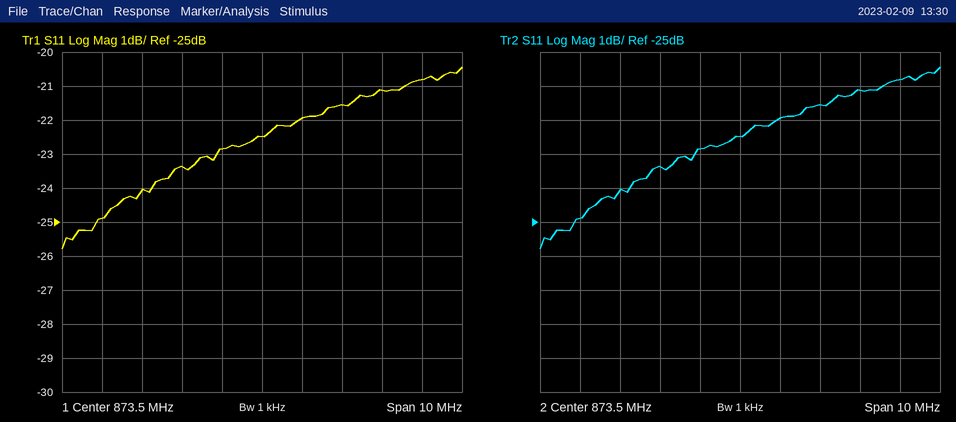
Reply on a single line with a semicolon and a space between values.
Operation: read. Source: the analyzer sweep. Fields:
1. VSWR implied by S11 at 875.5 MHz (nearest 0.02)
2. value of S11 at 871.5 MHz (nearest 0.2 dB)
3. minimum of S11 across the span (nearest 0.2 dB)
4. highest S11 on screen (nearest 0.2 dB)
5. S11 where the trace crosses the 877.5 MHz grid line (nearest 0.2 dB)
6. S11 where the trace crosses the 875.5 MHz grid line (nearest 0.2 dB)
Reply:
1.18; -23.4 dB; -25.8 dB; -20.4 dB; -20.8 dB; -21.6 dB
